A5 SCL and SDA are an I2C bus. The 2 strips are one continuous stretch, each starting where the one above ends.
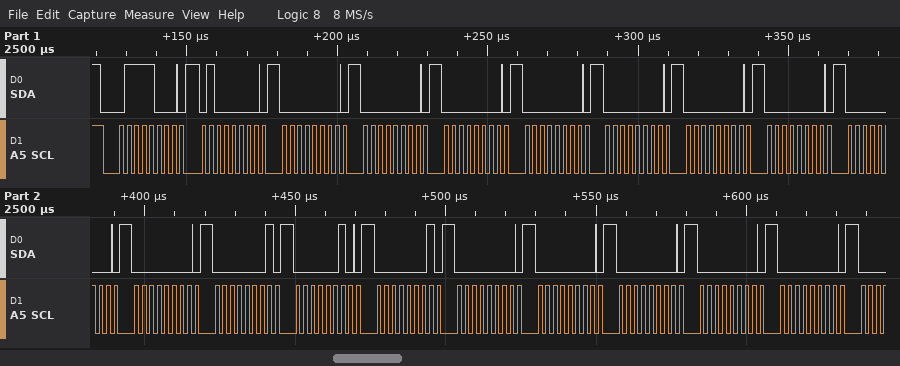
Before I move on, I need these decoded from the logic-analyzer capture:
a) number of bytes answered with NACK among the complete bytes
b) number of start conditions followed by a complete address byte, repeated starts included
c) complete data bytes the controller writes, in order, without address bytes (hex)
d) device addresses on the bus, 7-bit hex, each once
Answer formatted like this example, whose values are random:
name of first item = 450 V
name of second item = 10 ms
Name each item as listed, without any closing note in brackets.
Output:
number of bytes answered with NACK among the complete bytes = 0
number of start conditions followed by a complete address byte, repeated starts included = 1
complete data bytes the controller writes, in order, without address bytes = 40 00 00 00 00 00 00 00 00 00 01 02 01 00 00 00 00 00
device addresses on the bus, 7-bit hex, each once = 0x3C
